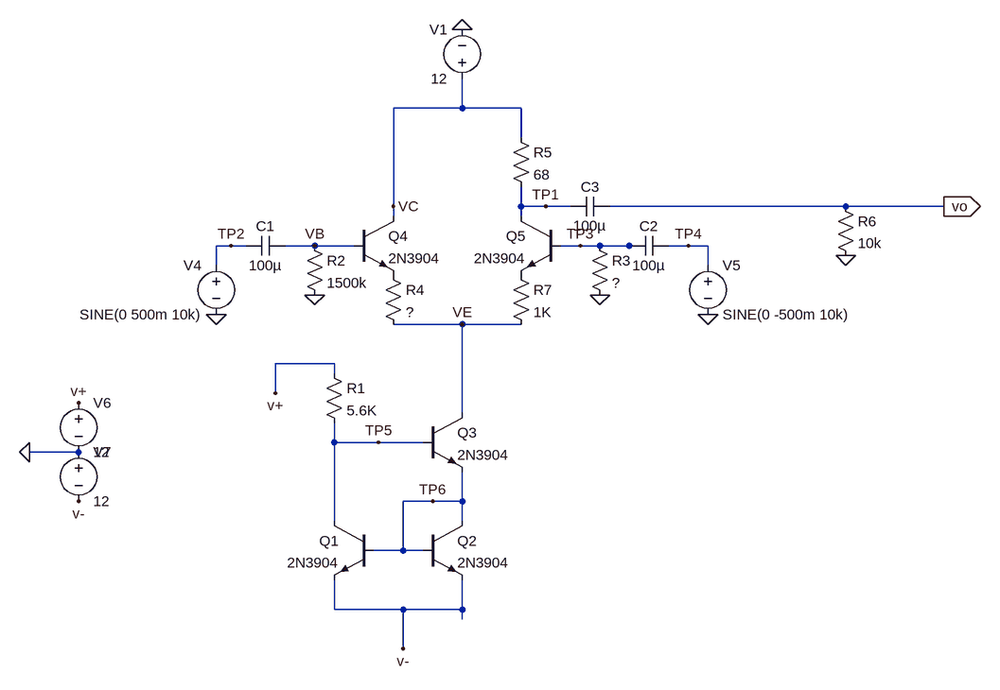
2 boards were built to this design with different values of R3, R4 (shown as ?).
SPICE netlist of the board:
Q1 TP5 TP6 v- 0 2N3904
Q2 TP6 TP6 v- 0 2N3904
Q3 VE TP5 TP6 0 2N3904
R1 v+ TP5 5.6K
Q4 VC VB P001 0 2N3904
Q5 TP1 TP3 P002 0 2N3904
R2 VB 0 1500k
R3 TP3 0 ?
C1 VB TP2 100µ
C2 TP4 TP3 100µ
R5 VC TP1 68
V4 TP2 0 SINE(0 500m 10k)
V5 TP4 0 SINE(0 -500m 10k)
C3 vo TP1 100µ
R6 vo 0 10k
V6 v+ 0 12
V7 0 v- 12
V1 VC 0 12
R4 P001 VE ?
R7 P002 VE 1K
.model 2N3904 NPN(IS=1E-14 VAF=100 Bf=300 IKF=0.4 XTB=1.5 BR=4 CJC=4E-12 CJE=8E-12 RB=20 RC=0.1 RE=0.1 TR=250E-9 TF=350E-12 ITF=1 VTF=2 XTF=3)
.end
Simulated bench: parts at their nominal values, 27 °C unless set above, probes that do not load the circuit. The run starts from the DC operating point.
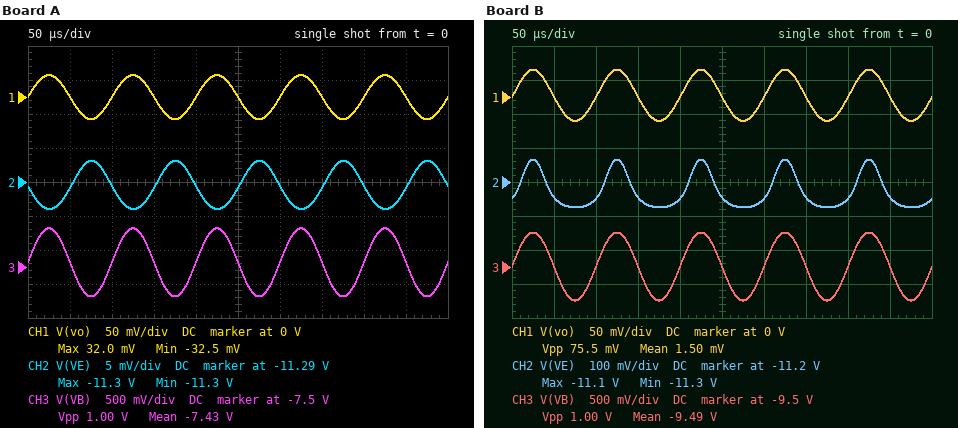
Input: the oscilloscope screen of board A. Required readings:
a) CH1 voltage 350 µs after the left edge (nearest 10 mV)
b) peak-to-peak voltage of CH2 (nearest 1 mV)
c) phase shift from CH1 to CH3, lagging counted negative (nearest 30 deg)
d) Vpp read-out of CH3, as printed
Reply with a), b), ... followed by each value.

a) 0 V
b) 7 mV
c) 0 deg
d) 1.00 V
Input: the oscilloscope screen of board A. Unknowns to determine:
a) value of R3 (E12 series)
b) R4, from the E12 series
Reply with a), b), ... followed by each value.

a) 3.9 MΩ
b) 1.8 kΩ
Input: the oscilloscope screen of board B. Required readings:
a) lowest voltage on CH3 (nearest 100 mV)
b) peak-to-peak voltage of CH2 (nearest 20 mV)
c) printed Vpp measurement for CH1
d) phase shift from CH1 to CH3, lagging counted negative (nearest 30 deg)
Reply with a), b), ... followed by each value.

a) -10.0 V
b) 140 mV
c) 75.5 mV
d) 0 deg
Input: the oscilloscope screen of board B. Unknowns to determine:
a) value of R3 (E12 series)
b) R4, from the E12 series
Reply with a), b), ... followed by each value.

a) 2.2 MΩ
b) 470 Ω
